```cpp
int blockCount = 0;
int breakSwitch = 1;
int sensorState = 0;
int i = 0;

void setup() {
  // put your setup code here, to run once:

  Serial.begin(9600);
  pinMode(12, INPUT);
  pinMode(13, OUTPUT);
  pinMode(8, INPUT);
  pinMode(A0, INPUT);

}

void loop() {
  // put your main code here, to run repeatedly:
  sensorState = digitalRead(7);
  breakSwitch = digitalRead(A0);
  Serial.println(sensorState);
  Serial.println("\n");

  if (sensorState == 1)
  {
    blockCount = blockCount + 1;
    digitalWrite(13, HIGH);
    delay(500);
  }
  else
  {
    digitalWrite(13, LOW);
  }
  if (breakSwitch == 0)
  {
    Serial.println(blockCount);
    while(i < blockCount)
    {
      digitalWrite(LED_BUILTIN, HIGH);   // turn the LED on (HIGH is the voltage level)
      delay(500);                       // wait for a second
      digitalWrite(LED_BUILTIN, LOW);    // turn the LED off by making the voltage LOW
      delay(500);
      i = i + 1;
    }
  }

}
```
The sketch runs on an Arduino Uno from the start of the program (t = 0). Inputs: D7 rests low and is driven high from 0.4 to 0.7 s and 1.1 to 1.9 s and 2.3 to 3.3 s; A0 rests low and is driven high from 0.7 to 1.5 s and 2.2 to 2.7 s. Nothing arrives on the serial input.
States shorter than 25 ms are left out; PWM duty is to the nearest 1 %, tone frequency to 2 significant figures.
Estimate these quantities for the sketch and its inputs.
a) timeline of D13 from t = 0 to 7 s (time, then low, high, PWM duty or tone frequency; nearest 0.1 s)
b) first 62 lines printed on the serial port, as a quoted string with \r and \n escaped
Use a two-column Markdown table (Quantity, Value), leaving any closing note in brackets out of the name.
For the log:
| Quantity | Value |
|---|---|
| timeline of D13 from t = 0 to 7 s | 0 s low; 0.4 s high; 1.4 s low; 2.3 s high; 3.8 s low; 4.3 s high; 4.8 s low |
| first 62 lines printed on the serial port, as a quoted string with \r and \n escaped | "0\r\n\n\r\n0\r\n0\r\n\n\r\n0\r\n0\r\n\n\r\n0\r\n0\r\n\n\r\n0\r\n0\r\n\n\r\n0\r\n0\r\n\n\r\n0\r\n0\r\n\n\r\n0\r\n0\r\n\n\r\n0\r\n0\r\n\n\r\n0\r\n0\r\n\n\r\n0\r\n0\r\n\n\r\n0\r\n0\r\n\n\r\n0\r\n0\r\n\n\r\n0\r\n0\r\n\n\r\n0\r\n0\r\n\n\r\n0\r\n0\r\n\n" |
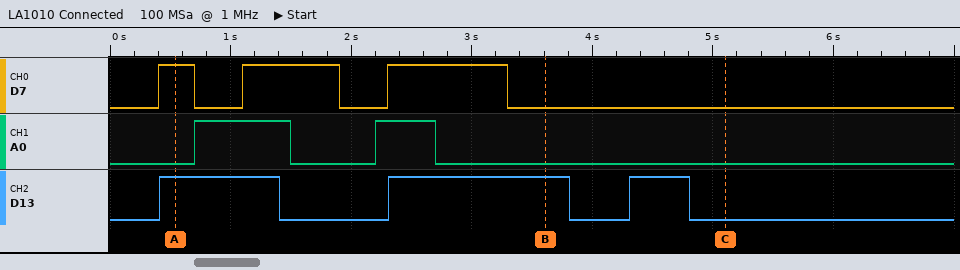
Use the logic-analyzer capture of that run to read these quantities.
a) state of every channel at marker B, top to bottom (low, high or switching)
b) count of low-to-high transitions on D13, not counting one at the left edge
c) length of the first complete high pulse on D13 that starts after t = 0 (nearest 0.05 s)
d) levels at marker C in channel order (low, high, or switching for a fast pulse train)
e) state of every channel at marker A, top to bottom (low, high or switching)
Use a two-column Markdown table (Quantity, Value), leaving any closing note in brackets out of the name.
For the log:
| Quantity | Value |
|---|---|
| state of every channel at marker B, top to bottom | D7 low, A0 low, D13 high |
| count of low-to-high transitions on D13, not counting one at the left edge | 3 |
| length of the first complete high pulse on D13 that starts after t = 0 | 1.00 s |
| levels at marker C in channel order | D7 low, A0 low, D13 low |
| state of every channel at marker A, top to bottom | D7 high, A0 low, D13 high |
